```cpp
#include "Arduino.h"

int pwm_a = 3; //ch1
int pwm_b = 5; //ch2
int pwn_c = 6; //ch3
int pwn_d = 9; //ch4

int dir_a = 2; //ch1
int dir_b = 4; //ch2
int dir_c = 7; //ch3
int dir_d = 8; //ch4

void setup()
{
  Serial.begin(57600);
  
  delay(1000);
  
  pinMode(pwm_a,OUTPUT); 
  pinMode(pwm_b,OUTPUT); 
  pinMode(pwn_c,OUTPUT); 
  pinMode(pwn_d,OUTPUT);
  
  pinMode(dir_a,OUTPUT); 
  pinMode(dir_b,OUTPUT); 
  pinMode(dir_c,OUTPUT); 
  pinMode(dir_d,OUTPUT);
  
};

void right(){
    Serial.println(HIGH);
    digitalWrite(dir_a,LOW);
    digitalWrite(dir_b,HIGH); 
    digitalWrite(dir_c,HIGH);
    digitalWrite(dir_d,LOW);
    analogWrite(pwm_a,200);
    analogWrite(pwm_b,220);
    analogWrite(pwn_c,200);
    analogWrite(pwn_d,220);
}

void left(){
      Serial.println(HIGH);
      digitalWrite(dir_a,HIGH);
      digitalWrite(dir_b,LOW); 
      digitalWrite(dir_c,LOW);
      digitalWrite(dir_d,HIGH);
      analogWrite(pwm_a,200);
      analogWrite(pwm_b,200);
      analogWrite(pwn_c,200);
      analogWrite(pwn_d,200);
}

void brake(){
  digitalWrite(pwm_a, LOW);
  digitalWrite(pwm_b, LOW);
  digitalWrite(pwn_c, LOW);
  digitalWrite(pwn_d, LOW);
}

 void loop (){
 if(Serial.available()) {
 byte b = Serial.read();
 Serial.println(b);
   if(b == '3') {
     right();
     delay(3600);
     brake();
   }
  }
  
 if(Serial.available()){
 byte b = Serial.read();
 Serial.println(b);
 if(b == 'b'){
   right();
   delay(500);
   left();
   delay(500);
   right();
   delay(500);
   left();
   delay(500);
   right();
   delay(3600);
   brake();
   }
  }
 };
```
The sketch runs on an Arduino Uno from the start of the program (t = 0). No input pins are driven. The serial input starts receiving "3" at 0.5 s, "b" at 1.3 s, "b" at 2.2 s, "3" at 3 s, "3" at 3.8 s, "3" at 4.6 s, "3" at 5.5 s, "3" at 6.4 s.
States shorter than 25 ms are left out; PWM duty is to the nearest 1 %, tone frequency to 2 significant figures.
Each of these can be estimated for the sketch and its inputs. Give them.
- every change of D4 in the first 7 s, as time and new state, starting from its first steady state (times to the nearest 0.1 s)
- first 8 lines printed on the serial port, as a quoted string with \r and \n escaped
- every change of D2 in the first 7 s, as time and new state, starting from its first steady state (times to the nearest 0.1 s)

1 s high; 5.1 s low; 5.6 s high; 6.1 s low; 6.6 s high
"51\r\n1\r\n98\r\n1\r\n1\r\n1\r\n1\r\n1\r\n"
1 s low; 5.1 s high; 5.6 s low; 6.1 s high; 6.6 s low
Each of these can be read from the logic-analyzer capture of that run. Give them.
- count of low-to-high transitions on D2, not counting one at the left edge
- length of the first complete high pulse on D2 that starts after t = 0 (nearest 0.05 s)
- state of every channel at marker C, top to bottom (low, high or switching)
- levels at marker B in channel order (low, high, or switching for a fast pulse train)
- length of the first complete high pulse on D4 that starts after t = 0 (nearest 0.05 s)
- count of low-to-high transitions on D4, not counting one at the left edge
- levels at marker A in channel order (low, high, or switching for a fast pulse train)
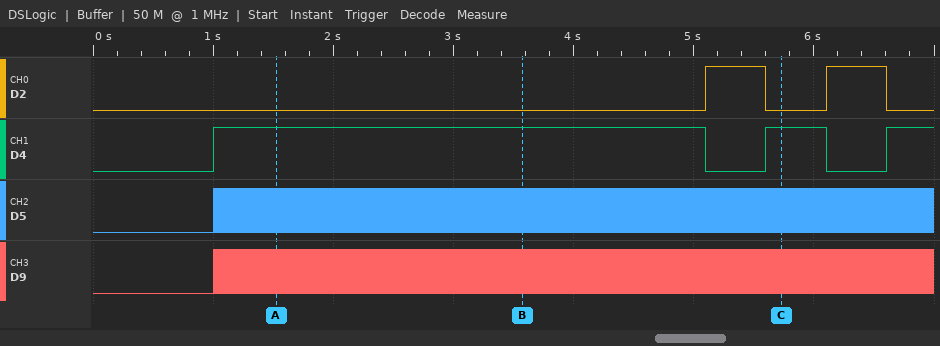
2
0.50 s
D2 low, D4 high, D5 switching, D9 switching
D2 low, D4 high, D5 switching, D9 switching
4.10 s
3
D2 low, D4 high, D5 switching, D9 switching
